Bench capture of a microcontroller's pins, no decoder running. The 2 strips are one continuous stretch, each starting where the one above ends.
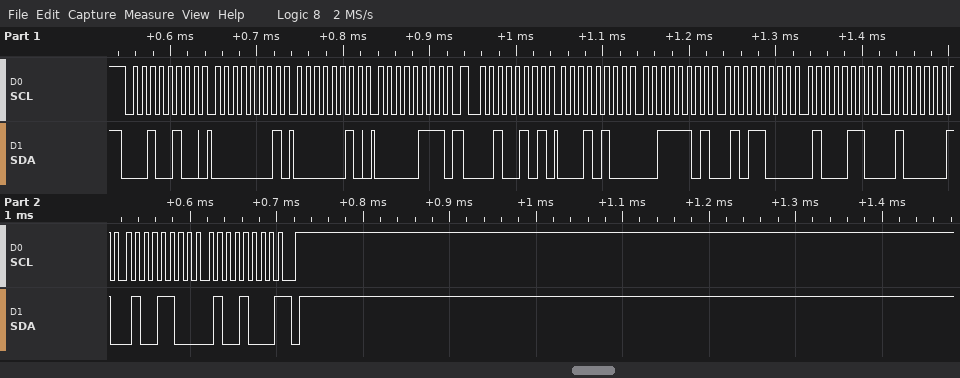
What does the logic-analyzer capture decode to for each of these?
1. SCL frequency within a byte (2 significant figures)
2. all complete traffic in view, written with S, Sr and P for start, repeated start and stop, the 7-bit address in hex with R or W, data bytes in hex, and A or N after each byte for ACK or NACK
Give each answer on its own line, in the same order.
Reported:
100 kHz
S 12W A 01 A 02 A 07 A Sr 12R A 14 A 3D A 58 A 46 A 41 A 4C A 48 N P
